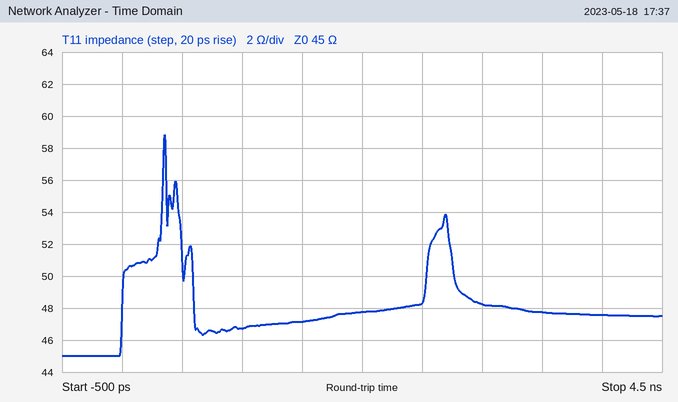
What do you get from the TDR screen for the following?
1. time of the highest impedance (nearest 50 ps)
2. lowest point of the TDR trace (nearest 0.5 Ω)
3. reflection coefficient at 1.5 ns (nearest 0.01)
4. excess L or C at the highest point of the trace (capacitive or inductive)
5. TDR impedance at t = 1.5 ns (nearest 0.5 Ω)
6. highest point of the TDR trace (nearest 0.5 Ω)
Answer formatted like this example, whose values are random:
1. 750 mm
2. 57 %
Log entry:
1. 350 ps
2. 45.0 Ω
3. +0.02
4. inductive
5. 47.0 Ω
6. 59.0 Ω
